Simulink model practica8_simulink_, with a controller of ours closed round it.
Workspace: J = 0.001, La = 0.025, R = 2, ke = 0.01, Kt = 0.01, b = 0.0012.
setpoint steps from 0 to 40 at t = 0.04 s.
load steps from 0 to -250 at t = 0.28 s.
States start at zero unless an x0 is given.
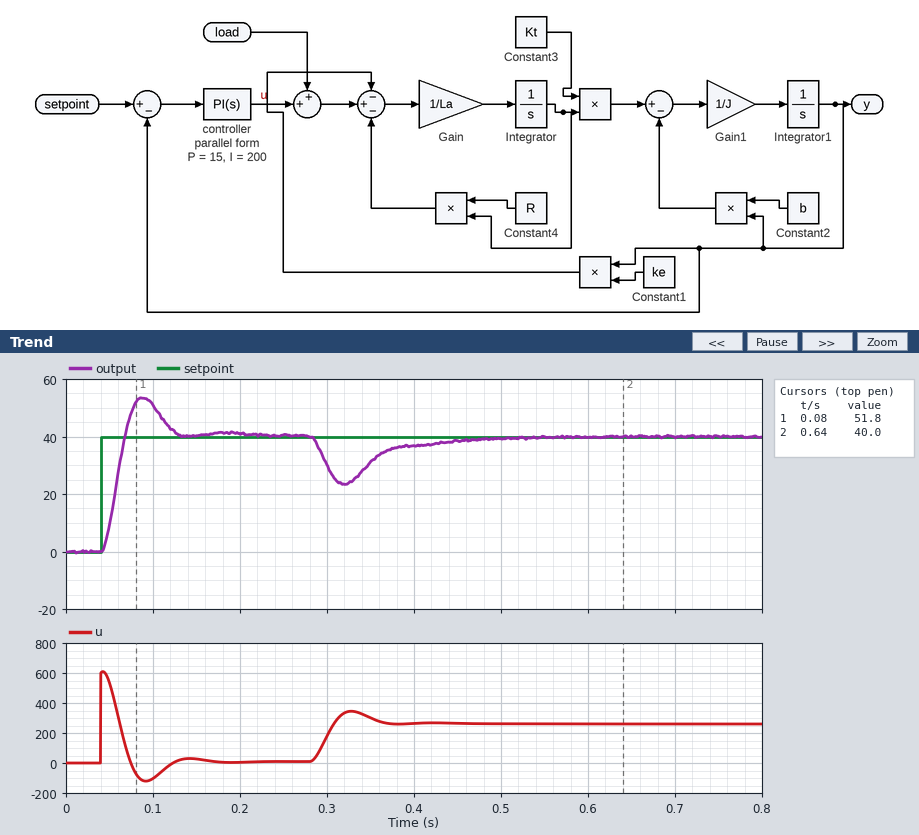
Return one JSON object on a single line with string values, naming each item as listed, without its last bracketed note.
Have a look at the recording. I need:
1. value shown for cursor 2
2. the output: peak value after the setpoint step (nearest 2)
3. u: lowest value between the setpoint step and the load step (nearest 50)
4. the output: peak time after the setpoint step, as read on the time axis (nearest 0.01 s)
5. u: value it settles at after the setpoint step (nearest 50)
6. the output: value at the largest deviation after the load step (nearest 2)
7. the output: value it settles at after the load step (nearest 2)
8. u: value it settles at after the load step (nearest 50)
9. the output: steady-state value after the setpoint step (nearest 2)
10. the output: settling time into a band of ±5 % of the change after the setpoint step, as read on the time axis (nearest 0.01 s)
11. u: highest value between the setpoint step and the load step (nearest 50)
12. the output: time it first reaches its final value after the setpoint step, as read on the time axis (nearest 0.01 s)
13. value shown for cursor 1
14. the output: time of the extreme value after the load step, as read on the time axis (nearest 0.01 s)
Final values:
{"value shown for cursor 2": "40.0", "the output: peak value after the setpoint step": "54", "u: lowest value between the setpoint step and the load step": "-100", "the output: peak time after the setpoint step, as read on the time axis": "0.09 s", "u: value it settles at after the setpoint step": "0", "the output: value at the largest deviation after the load step": "24", "the output: value it settles at after the load step": "40", "u: value it settles at after the load step": "250", "the output: steady-state value after the setpoint step": "40", "the output: settling time into a band of ±5 % of the change after the setpoint step, as read on the time axis": "0.12 s", "u: highest value between the setpoint step and the load step": "600", "the output: time it first reaches its final value after the setpoint step, as read on the time axis": "0.07 s", "value shown for cursor 1": "51.8", "the output: time of the extreme value after the load step, as read on the time axis": "0.32 s"}
